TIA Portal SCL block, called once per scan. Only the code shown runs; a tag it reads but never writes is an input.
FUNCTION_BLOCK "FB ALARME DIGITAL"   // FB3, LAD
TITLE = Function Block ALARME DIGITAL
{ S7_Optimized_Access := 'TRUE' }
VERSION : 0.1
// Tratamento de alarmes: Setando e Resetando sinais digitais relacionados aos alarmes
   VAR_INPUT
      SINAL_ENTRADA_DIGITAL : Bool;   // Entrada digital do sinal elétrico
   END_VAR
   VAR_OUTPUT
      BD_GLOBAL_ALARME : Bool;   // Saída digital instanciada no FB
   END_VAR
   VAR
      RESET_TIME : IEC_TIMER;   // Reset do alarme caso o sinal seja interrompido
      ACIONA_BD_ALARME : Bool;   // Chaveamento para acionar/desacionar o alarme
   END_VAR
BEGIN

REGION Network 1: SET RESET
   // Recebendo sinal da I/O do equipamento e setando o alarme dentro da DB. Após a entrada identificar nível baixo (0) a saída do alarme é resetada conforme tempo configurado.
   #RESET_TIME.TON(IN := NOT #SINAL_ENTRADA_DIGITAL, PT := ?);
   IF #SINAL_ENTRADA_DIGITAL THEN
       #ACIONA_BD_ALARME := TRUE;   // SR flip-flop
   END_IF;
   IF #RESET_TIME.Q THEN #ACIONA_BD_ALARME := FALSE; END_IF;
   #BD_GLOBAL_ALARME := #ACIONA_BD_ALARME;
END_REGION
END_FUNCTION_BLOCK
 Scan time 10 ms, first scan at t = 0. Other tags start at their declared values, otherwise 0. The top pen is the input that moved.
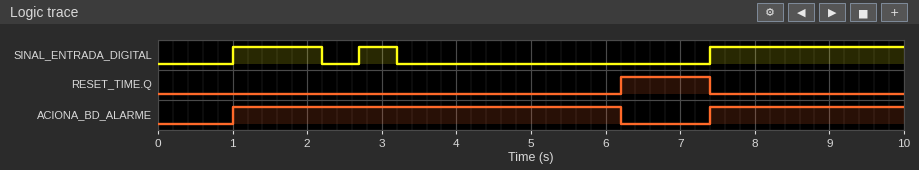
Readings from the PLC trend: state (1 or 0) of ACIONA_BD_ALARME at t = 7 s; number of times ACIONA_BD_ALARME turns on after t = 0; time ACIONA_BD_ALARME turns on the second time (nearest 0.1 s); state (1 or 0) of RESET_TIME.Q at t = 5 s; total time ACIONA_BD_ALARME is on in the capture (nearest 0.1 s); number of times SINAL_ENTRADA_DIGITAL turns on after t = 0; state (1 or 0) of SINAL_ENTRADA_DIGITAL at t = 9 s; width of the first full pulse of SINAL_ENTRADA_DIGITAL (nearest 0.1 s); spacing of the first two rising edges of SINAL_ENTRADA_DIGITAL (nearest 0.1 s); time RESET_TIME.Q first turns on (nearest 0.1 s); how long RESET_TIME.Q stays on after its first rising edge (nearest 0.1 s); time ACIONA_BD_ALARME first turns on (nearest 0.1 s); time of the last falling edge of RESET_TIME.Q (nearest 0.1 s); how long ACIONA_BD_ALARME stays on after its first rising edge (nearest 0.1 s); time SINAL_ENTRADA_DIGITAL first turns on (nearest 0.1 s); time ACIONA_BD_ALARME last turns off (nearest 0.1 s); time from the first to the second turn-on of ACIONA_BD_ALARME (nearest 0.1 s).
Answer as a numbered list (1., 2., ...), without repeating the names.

1. 0
2. 2
3. 7.4 s
4. 0
5. 7.8 s
6. 3
7. 1
8. 1.2 s
9. 1.7 s
10. 6.2 s
11. 1.2 s
12. 1.0 s
13. 7.4 s
14. 5.2 s
15. 1.0 s
16. 6.2 s
17. 6.4 s
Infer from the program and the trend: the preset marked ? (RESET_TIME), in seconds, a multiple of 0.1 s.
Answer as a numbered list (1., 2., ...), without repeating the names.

1. 3.0 s
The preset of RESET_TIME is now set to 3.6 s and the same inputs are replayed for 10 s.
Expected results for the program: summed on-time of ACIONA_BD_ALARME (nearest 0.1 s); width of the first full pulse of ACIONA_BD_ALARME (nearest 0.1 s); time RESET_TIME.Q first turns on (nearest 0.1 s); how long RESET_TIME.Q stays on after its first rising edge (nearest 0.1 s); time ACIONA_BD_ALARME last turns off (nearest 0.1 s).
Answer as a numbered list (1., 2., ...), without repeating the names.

1. 8.4 s
2. 5.8 s
3. 6.8 s
4. 0.6 s
5. 6.8 s
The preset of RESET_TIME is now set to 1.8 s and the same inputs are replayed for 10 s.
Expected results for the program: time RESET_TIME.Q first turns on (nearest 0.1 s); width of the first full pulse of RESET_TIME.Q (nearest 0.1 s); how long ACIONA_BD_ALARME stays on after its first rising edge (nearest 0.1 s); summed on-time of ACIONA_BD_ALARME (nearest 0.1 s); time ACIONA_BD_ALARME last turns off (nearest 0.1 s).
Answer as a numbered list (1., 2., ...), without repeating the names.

1. 5.0 s
2. 2.4 s
3. 4.0 s
4. 6.6 s
5. 5.0 s
